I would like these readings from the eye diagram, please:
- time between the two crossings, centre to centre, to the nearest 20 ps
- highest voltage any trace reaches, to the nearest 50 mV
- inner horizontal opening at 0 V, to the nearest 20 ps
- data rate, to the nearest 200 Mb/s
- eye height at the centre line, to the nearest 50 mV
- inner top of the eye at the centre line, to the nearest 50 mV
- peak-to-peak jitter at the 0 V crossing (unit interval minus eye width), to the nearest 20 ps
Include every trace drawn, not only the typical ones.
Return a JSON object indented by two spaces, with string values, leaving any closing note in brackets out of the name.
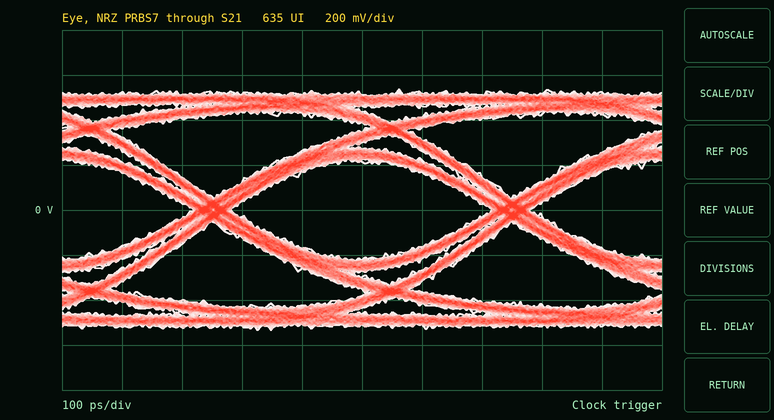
{
  "time between the two crossings, centre to centre, to the nearest 20 ps": "500 ps",
  "highest voltage any trace reaches, to the nearest 50 mV": "550 mV",
  "inner horizontal opening at 0 V, to the nearest 20 ps": "440 ps",
  "data rate, to the nearest 200 Mb/s": "2.0 Gb/s",
  "eye height at the centre line, to the nearest 50 mV": "450 mV",
  "inner top of the eye at the centre line, to the nearest 50 mV": "200 mV",
  "peak-to-peak jitter at the 0 V crossing (unit interval minus eye width), to the nearest 20 ps": "60 ps"
}
